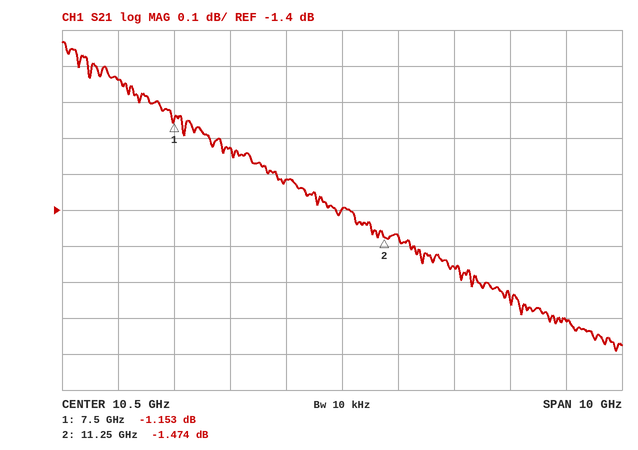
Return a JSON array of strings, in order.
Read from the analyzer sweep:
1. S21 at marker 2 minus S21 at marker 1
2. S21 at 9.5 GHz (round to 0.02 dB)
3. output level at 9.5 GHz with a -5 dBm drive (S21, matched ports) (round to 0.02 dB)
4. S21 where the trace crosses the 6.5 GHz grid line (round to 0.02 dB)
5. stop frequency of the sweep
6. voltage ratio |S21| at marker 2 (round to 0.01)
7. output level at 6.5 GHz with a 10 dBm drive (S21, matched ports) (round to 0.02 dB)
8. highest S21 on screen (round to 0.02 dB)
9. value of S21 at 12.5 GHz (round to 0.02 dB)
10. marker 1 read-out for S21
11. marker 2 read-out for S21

["-0.321 dB", "-1.32 dB", "-6.32 dBm", "-1.04 dB", "15.5 GHz", "0.84", "8.96 dBm", "-0.94 dB", "-1.56 dB", "-1.153 dB", "-1.474 dB"]
